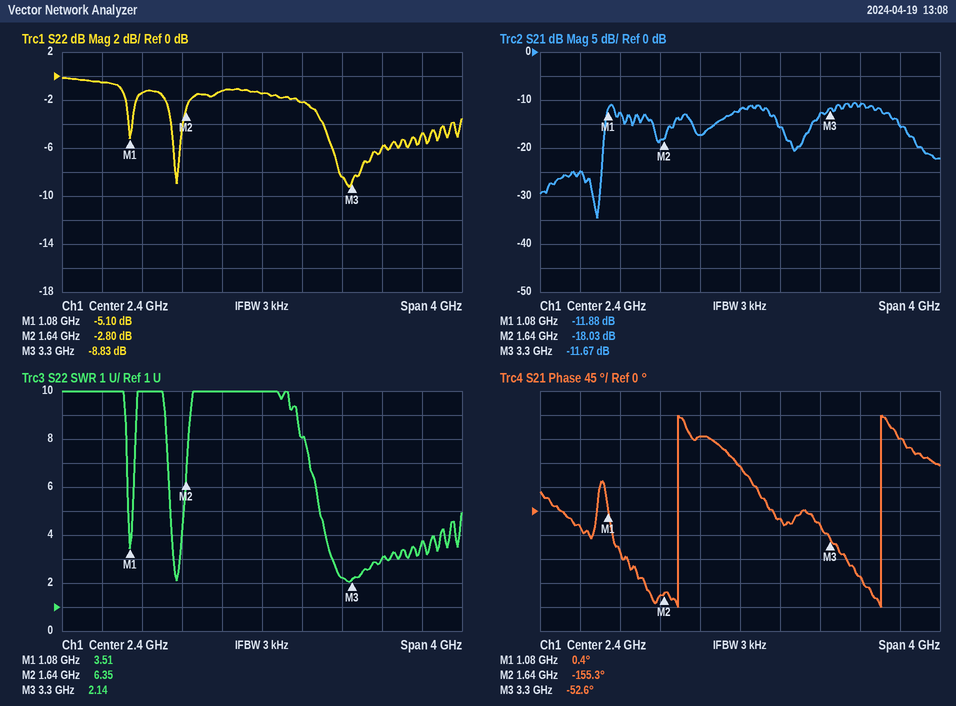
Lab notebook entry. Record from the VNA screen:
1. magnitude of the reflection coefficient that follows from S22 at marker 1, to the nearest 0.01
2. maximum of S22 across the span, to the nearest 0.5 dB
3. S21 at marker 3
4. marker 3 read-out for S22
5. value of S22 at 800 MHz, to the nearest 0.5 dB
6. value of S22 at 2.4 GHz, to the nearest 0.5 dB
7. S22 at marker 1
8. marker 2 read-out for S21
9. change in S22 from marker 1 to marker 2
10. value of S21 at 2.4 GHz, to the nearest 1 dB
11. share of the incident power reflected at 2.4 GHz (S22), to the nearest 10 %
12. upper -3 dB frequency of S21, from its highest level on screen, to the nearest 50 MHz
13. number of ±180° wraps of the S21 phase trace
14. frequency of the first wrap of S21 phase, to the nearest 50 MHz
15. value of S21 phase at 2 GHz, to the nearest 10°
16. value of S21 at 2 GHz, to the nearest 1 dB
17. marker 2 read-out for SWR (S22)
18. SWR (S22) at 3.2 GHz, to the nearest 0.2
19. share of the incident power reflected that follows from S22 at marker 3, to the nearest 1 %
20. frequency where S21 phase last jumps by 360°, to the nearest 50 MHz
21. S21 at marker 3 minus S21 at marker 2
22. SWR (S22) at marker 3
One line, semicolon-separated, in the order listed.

0.56; 0.0 dB; -11.67 dB; -8.83 dB; -0.5 dB; -1.5 dB; -5.10 dB; -18.03 dB; 2.30 dB; -12 dB; 70 %; 3.90 GHz; 2; 1.80 GHz; 140°; -17 dB; 6.35; 2.2; 13 %; 3.80 GHz; 6.36 dB; 2.14
